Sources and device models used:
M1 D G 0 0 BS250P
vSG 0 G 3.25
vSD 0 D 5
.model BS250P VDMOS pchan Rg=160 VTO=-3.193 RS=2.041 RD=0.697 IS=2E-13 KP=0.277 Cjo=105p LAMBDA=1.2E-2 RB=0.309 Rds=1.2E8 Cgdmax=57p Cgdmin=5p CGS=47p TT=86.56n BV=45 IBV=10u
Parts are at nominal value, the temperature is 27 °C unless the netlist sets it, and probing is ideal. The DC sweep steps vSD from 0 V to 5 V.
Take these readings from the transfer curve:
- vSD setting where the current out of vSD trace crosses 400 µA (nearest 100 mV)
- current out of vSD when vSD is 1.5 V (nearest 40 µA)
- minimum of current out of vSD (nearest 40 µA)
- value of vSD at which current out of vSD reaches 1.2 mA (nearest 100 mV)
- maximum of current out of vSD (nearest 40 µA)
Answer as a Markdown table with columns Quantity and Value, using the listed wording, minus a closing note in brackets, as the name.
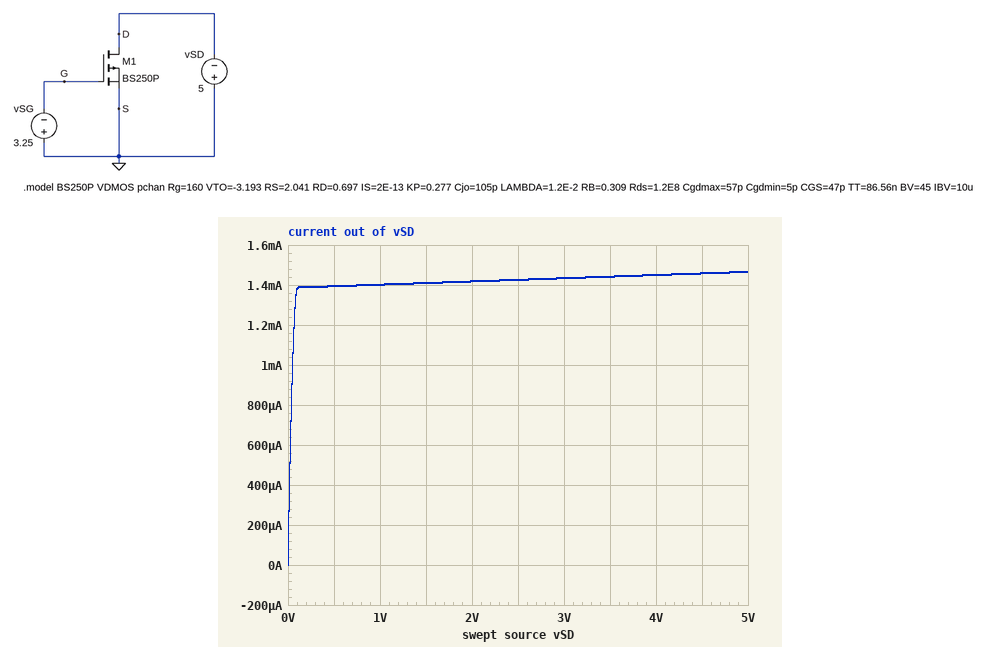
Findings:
| Quantity | Value |
|---|---|
| vSD setting where the current out of vSD trace crosses 400 µA | 0 V |
| current out of vSD when vSD is 1.5 V | 1.40 mA |
| minimum of current out of vSD | 0 A |
| value of vSD at which current out of vSD reaches 1.2 mA | 100 mV |
| maximum of current out of vSD | 1.48 mA |
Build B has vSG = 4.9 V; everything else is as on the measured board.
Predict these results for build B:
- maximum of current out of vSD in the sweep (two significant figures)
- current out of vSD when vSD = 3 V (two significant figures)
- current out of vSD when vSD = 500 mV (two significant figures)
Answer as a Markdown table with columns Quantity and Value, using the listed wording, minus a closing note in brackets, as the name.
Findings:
| Quantity | Value |
|---|---|
| maximum of current out of vSD in the sweep | 230 mA |
| current out of vSD when vSD = 3 V | 220 mA |
| current out of vSD when vSD = 500 mV | 94 mA |
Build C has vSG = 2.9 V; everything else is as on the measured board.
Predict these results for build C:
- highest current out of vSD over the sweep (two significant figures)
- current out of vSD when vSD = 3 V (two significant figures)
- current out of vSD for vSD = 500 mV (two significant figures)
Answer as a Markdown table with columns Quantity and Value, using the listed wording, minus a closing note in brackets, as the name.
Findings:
| Quantity | Value |
|---|---|
| highest current out of vSD over the sweep | 4.0 µA |
| current out of vSD when vSD = 3 V | 3.9 µA |
| current out of vSD for vSD = 500 mV | 3.8 µA |
